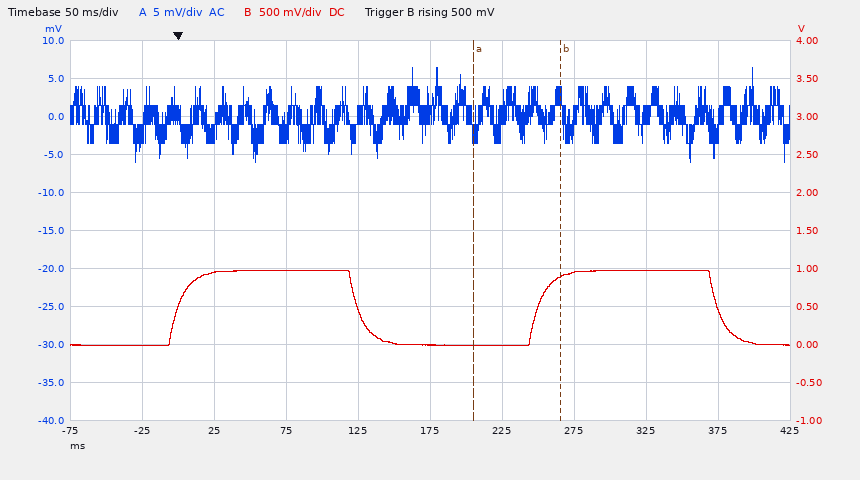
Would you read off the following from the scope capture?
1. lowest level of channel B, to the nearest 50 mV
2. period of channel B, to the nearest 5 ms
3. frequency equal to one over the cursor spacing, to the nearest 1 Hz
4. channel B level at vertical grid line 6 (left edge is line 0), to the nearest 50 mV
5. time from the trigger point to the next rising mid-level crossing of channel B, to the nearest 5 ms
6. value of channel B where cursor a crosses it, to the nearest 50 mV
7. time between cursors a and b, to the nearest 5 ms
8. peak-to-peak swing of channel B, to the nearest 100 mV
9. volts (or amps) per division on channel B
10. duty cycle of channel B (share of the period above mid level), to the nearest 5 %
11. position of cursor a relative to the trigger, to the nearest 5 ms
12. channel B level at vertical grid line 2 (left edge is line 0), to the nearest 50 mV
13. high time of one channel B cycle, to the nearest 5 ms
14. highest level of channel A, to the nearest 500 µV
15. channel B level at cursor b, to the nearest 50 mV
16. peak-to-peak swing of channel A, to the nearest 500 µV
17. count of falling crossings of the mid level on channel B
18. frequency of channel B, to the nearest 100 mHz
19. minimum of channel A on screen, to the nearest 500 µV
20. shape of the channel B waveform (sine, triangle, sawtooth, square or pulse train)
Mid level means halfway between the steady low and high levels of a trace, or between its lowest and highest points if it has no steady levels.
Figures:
0 mV
250 ms
17 Hz
0 mV
250 ms
0 mV
60 ms
1.00 V
500 mV
50 %
+205 ms
950 mV
125 ms
6.5 mV
900 mV
12.5 mV
2
4.0 Hz
-6.0 mV
square
